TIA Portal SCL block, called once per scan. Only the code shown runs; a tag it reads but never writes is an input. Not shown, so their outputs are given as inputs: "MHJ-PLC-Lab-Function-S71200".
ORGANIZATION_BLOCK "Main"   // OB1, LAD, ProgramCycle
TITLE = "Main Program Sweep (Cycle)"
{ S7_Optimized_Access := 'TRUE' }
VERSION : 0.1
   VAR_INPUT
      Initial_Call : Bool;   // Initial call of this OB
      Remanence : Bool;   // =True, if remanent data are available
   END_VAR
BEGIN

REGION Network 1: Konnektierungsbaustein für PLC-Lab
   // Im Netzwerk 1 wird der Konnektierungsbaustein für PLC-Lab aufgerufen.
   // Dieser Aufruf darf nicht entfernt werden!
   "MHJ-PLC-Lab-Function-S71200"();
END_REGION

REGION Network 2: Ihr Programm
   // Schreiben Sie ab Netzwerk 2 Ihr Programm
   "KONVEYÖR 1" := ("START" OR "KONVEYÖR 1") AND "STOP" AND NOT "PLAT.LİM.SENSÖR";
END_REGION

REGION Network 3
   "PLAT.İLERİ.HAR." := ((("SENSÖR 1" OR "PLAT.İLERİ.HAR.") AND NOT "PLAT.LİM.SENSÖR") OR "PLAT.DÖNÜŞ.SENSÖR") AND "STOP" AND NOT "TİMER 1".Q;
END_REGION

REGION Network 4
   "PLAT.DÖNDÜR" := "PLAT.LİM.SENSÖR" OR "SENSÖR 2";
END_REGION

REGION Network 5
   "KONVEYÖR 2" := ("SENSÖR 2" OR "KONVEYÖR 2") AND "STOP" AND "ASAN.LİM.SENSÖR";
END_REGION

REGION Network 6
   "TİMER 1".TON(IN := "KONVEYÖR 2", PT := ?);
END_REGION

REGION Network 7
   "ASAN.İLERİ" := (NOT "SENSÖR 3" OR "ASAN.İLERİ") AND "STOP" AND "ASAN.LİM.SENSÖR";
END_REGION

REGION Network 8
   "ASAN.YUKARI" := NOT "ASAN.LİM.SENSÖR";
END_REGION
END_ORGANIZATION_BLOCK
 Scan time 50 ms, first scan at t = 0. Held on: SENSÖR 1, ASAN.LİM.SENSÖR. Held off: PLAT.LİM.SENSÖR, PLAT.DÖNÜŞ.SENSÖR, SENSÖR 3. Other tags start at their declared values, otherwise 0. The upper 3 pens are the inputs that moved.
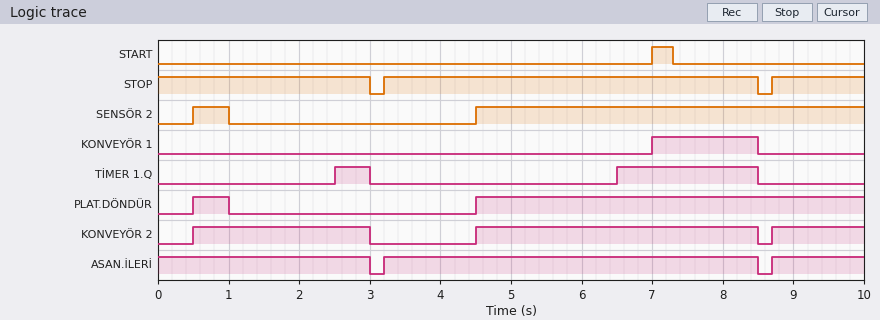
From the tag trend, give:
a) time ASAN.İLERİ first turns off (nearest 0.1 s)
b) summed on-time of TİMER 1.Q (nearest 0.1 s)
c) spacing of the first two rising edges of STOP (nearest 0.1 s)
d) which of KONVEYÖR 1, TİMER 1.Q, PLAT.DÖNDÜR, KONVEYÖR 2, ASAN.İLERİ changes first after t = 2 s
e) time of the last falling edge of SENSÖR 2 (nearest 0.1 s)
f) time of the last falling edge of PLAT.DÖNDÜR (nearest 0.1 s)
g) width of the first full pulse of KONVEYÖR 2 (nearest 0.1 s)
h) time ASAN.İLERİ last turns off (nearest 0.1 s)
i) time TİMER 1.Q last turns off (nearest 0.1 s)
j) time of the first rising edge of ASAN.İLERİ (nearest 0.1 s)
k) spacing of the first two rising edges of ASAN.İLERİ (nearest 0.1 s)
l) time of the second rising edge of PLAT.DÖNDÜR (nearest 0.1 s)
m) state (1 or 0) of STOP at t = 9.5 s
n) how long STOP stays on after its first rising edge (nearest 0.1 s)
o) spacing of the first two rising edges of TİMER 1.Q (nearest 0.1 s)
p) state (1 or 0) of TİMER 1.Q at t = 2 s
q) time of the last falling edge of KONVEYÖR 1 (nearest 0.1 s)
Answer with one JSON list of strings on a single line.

["3.0 s", "2.5 s", "5.5 s", "TİMER 1.Q", "1.0 s", "1.0 s", "2.5 s", "8.5 s", "8.5 s", "3.2 s", "5.5 s", "4.5 s", "1", "5.3 s", "4.0 s", "0", "8.5 s"]
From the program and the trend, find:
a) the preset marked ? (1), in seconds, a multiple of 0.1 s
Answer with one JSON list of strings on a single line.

["2.0 s"]
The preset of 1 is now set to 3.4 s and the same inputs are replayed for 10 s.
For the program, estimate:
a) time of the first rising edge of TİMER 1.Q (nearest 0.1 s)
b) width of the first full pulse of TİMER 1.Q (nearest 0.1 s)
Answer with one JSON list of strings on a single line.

["7.9 s", "0.6 s"]
